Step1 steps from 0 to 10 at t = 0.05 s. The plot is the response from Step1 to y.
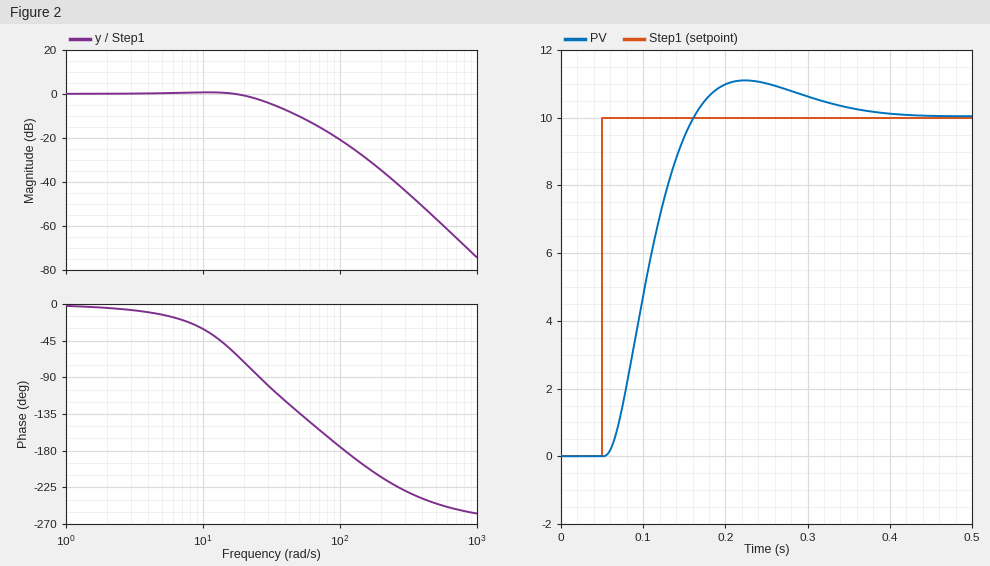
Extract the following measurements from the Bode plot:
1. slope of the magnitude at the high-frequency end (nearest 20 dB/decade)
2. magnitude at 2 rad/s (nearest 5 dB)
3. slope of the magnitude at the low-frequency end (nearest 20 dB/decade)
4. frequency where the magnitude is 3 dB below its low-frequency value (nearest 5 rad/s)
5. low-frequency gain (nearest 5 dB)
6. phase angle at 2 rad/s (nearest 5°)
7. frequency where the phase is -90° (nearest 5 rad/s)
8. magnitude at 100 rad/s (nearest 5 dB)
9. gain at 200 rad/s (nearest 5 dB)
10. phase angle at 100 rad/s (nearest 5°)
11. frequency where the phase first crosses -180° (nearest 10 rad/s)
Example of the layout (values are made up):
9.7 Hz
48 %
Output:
-60 dB/decade
0 dB
0 dB/decade
25 rad/s
0 dB
-5°
25 rad/s
-20 dB
-35 dB
-175°
110 rad/s
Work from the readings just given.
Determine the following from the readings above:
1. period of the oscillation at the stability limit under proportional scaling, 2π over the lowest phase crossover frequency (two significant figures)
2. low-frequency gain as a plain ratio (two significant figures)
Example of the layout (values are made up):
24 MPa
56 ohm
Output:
0.057 s
1.0
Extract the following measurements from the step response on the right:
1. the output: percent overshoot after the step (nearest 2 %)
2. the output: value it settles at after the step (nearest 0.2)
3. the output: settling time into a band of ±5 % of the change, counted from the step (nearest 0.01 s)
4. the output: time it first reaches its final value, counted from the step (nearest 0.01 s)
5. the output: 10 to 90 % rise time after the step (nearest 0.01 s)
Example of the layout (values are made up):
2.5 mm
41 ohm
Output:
10 %
10.0
0.26 s
0.11 s
0.07 s
